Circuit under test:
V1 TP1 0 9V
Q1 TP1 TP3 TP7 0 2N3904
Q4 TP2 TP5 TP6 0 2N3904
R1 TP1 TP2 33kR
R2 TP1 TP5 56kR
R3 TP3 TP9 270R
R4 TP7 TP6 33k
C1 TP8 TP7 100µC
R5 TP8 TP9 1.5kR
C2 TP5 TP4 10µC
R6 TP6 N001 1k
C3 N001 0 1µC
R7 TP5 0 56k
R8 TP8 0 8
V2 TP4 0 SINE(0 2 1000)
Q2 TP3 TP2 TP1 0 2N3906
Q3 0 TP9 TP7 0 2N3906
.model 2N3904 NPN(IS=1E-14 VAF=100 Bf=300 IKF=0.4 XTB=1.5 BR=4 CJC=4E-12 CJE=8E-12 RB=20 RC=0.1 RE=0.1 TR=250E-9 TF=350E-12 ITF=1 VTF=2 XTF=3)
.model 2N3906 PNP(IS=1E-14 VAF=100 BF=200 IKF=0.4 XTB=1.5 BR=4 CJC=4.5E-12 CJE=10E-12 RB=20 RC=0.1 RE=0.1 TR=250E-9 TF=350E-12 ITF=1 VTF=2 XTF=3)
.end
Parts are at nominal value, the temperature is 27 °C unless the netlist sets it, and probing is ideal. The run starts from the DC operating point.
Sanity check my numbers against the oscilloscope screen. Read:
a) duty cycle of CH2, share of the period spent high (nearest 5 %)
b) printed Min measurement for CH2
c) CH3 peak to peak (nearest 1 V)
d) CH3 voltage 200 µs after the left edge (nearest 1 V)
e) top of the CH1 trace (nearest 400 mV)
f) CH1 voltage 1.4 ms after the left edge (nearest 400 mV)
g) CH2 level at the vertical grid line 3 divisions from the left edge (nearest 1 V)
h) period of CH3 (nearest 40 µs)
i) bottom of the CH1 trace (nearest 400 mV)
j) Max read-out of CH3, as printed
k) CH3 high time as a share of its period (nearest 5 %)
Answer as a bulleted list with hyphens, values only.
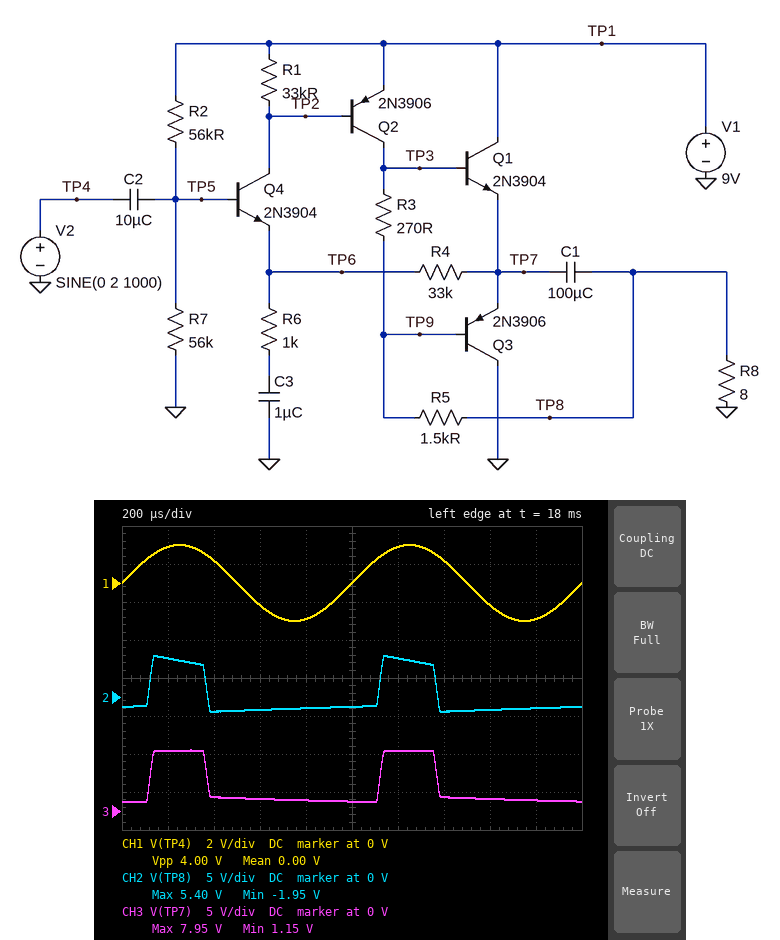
- 25 %
- -1.95 V
- 7 V
- 8 V
- 2.0 V
- 1.2 V
- -2 V
- 1.00 ms
- -2.0 V
- 7.95 V
- 25 %
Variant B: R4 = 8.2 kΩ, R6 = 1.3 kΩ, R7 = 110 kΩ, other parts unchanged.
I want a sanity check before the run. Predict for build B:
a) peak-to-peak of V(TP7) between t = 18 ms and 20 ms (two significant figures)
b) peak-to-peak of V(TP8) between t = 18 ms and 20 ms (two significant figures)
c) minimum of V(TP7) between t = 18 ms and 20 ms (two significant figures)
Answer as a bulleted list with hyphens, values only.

- 6.2 V
- 6.7 V
- 1.8 V
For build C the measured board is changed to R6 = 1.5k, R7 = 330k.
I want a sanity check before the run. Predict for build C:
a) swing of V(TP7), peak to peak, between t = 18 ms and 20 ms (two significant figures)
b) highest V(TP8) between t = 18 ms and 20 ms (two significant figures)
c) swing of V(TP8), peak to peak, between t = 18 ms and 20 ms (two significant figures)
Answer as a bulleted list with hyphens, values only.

- 7.0 V
- 6.0 V
- 7.3 V
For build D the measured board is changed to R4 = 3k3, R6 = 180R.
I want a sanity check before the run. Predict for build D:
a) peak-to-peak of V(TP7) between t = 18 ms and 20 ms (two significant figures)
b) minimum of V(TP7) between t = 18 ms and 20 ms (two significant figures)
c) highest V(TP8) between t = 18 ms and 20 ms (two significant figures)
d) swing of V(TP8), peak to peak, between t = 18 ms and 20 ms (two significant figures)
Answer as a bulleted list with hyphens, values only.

- 6.7 V
- 1.4 V
- 5.0 V
- 7.2 V
